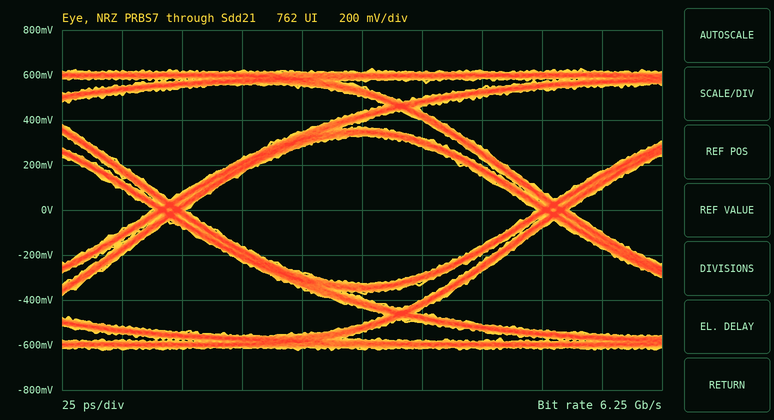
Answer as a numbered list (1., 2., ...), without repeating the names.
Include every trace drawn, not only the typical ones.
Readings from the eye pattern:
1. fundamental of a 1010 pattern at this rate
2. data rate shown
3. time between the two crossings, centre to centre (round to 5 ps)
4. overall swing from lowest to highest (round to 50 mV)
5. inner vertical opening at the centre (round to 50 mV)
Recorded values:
1. 3.125 GHz
2. 6.25 Gb/s
3. 160 ps
4. 1.25 V
5. 650 mV
